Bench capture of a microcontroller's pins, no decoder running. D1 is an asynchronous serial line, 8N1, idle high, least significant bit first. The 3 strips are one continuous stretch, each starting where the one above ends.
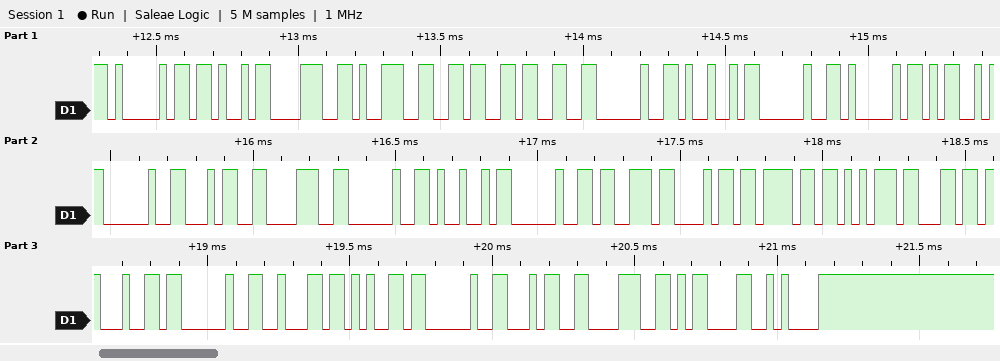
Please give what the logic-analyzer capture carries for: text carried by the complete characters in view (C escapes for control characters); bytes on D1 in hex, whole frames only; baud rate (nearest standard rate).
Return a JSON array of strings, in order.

["\"AK8963 I AM 48 I should be 48\\r\\n\"", "41 4B 38 39 36 33 20 49 20 41 4D 20 34 38 20 49 20 73 68 6F 75 6C 64 20 62 65 20 34 38 0D 0A", "38400 baud"]
